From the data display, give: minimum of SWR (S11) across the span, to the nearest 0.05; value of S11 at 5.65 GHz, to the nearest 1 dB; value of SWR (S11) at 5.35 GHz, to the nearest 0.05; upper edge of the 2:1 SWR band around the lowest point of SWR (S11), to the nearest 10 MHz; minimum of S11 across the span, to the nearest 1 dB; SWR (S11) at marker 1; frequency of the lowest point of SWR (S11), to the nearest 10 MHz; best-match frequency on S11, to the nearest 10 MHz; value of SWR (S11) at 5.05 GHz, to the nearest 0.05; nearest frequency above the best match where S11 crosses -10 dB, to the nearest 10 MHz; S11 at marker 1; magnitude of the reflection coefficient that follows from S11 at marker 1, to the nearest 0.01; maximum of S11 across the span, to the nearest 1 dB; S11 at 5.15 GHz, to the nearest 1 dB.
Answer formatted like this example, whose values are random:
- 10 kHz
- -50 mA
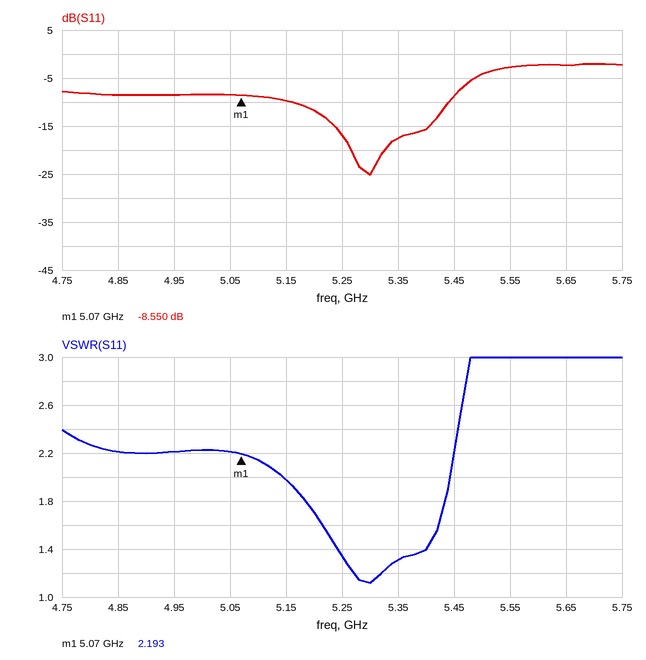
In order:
- 1.10
- -2 dB
- 1.30
- 5.44 GHz
- -25 dB
- 2.193
- 5.30 GHz
- 5.30 GHz
- 2.20
- 5.44 GHz
- -8.550 dB
- 0.37
- -2 dB
- -10 dB
